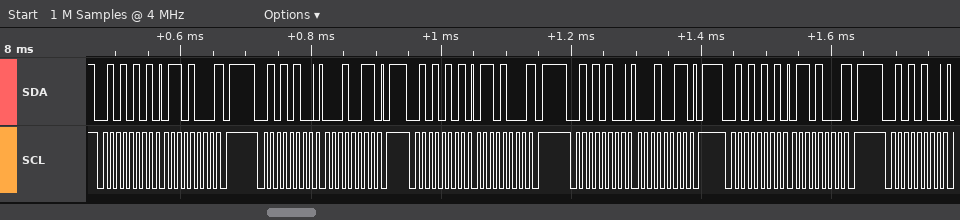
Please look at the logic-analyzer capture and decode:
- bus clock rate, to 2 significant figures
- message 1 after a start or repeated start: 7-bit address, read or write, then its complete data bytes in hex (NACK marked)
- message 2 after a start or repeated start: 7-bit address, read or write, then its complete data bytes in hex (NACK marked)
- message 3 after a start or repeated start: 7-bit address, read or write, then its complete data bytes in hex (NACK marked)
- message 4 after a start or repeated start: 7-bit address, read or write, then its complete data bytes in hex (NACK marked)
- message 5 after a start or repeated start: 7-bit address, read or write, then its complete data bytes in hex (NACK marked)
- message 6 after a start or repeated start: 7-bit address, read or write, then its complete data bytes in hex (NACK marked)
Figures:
100 kHz
0x2A read: 68 NACK
0x2A write: 13
0x2A read: 68 NACK
0x2A write: 13
0x2A read: 68 NACK
0x2A write
